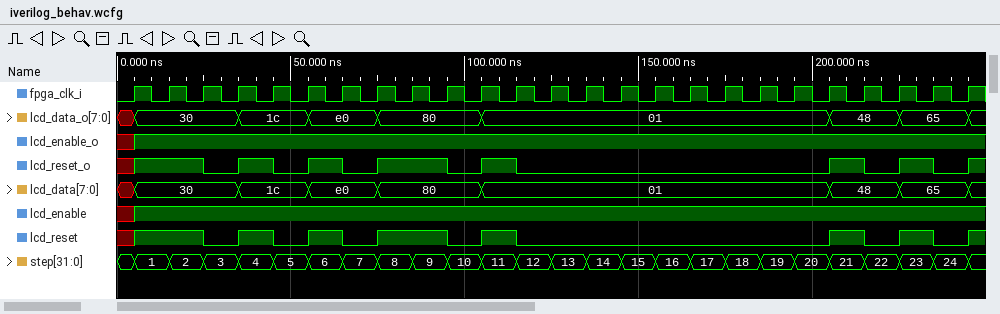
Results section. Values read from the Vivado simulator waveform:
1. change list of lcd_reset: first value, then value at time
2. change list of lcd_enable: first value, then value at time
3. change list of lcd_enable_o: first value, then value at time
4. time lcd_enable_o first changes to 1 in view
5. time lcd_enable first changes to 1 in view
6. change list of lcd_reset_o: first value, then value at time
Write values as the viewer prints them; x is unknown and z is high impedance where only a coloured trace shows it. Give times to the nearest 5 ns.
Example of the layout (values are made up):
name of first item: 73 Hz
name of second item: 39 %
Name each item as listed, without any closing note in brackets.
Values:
change list of lcd_reset: first value, then value at time: x, 1 at 5 ns, 0 at 25 ns, 1 at 35 ns, 0 at 45 ns, 1 at 55 ns, 0 at 65 ns, 1 at 75 ns, 0 at 95 ns, 1 at 105 ns, 0 at 115 ns, 1 at 205 ns, 0 at 215 ns, 1 at 225 ns, 0 at 235 ns, 1 at 245 ns
change list of lcd_enable: first value, then value at time: x, 1 at 5 ns
change list of lcd_enable_o: first value, then value at time: x, 1 at 5 ns
time lcd_enable_o first changes to 1 in view: 5 ns
time lcd_enable first changes to 1 in view: 5 ns
change list of lcd_reset_o: first value, then value at time: x, 1 at 5 ns, 0 at 25 ns, 1 at 35 ns, 0 at 45 ns, 1 at 55 ns, 0 at 65 ns, 1 at 75 ns, 0 at 95 ns, 1 at 105 ns, 0 at 115 ns, 1 at 205 ns, 0 at 215 ns, 1 at 225 ns, 0 at 235 ns, 1 at 245 ns
